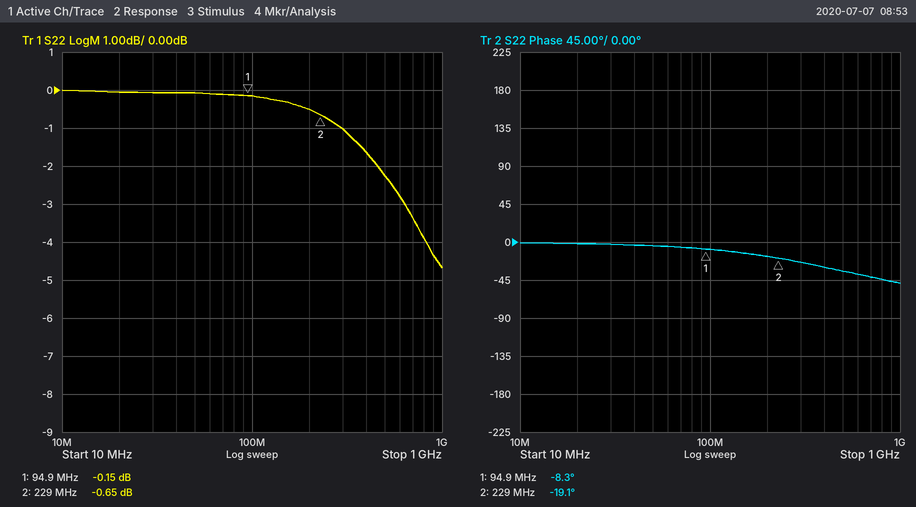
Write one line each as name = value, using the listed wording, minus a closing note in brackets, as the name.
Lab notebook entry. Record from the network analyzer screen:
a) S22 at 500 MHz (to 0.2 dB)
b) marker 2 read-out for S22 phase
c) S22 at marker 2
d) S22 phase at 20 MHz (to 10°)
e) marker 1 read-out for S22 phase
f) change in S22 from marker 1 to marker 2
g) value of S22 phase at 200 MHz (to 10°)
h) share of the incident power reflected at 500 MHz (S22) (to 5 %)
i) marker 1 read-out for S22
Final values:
S22 at 500 MHz = -2.2 dB
marker 2 read-out for S22 phase = -19.1°
S22 at marker 2 = -0.65 dB
S22 phase at 20 MHz = 0°
marker 1 read-out for S22 phase = -8.3°
change in S22 from marker 1 to marker 2 = -0.50 dB
value of S22 phase at 200 MHz = -20°
share of the incident power reflected at 500 MHz (S22) = 60 %
marker 1 read-out for S22 = -0.15 dB
